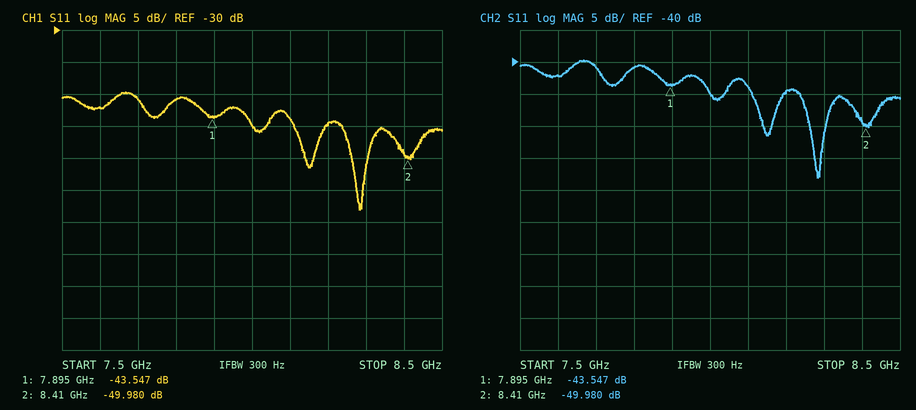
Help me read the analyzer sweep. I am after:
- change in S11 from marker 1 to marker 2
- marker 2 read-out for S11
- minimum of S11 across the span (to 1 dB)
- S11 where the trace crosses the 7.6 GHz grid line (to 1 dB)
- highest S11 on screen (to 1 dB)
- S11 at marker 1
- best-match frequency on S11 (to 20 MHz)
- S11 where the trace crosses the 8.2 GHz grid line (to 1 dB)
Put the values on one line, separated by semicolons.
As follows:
-6.433 dB; -49.980 dB; -58 dB; -42 dB; -40 dB; -43.547 dB; 8.28 GHz; -45 dB
